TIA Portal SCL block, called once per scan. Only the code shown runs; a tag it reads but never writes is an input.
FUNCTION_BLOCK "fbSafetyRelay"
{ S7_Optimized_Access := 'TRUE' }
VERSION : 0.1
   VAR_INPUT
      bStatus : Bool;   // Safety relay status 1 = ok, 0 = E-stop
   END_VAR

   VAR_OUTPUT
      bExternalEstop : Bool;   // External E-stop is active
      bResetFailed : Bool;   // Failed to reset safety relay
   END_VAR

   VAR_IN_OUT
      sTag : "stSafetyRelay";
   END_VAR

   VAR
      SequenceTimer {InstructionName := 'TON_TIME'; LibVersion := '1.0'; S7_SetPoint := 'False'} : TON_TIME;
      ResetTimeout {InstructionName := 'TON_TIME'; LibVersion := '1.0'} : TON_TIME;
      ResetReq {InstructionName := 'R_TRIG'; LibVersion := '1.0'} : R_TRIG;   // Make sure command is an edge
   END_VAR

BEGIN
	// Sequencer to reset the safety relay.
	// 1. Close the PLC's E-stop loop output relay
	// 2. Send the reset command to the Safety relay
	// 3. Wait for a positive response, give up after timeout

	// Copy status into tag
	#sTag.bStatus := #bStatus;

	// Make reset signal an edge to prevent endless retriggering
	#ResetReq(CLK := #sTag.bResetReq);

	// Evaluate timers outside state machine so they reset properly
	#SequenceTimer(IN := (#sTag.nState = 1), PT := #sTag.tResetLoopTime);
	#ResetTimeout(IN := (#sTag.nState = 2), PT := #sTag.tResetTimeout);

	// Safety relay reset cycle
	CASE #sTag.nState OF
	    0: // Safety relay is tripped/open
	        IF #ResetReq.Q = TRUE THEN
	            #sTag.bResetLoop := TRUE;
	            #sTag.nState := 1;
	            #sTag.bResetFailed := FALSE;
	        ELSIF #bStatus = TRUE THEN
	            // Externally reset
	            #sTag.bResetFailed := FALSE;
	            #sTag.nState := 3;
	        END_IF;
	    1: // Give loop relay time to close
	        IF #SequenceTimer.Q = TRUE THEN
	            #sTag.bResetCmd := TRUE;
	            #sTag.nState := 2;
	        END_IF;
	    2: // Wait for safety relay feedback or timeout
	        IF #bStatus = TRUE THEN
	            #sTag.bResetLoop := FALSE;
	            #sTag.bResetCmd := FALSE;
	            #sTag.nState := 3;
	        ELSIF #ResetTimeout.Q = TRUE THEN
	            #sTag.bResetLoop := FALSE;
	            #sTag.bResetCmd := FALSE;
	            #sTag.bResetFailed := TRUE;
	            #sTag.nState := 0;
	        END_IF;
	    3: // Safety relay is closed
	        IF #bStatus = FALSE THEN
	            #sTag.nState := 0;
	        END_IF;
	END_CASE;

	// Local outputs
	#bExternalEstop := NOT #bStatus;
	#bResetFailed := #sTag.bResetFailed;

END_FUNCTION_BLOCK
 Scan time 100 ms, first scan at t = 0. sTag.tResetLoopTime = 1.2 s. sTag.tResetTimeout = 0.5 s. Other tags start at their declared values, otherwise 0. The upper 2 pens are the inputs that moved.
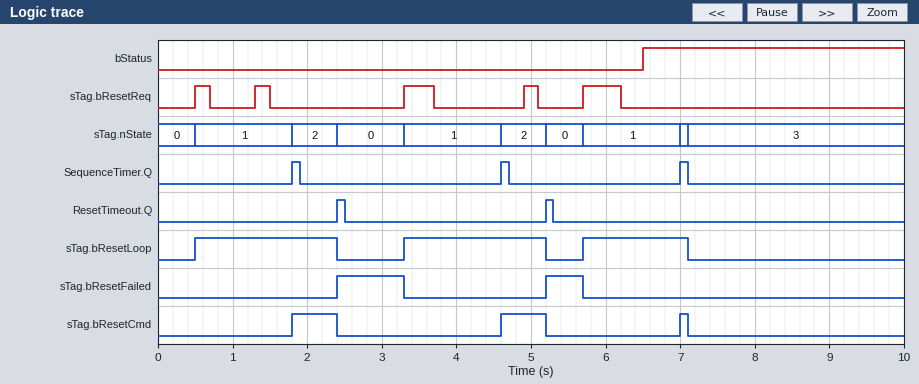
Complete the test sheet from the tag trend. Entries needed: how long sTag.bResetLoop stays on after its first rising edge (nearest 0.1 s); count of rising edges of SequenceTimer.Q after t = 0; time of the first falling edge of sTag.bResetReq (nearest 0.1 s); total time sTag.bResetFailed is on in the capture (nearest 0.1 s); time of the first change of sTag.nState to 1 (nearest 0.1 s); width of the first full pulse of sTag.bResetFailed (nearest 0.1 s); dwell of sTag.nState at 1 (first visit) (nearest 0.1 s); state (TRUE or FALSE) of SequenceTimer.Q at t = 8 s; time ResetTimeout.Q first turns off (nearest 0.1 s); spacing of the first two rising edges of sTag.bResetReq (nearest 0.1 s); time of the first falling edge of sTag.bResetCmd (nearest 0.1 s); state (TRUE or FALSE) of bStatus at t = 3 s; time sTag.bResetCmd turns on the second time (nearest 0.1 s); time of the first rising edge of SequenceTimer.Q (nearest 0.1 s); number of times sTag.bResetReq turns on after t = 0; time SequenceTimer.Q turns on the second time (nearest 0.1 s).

1.9 s
3
0.7 s
1.4 s
0.5 s
0.9 s
1.3 s
FALSE
2.5 s
0.8 s
2.4 s
FALSE
4.6 s
1.8 s
5
4.6 s
